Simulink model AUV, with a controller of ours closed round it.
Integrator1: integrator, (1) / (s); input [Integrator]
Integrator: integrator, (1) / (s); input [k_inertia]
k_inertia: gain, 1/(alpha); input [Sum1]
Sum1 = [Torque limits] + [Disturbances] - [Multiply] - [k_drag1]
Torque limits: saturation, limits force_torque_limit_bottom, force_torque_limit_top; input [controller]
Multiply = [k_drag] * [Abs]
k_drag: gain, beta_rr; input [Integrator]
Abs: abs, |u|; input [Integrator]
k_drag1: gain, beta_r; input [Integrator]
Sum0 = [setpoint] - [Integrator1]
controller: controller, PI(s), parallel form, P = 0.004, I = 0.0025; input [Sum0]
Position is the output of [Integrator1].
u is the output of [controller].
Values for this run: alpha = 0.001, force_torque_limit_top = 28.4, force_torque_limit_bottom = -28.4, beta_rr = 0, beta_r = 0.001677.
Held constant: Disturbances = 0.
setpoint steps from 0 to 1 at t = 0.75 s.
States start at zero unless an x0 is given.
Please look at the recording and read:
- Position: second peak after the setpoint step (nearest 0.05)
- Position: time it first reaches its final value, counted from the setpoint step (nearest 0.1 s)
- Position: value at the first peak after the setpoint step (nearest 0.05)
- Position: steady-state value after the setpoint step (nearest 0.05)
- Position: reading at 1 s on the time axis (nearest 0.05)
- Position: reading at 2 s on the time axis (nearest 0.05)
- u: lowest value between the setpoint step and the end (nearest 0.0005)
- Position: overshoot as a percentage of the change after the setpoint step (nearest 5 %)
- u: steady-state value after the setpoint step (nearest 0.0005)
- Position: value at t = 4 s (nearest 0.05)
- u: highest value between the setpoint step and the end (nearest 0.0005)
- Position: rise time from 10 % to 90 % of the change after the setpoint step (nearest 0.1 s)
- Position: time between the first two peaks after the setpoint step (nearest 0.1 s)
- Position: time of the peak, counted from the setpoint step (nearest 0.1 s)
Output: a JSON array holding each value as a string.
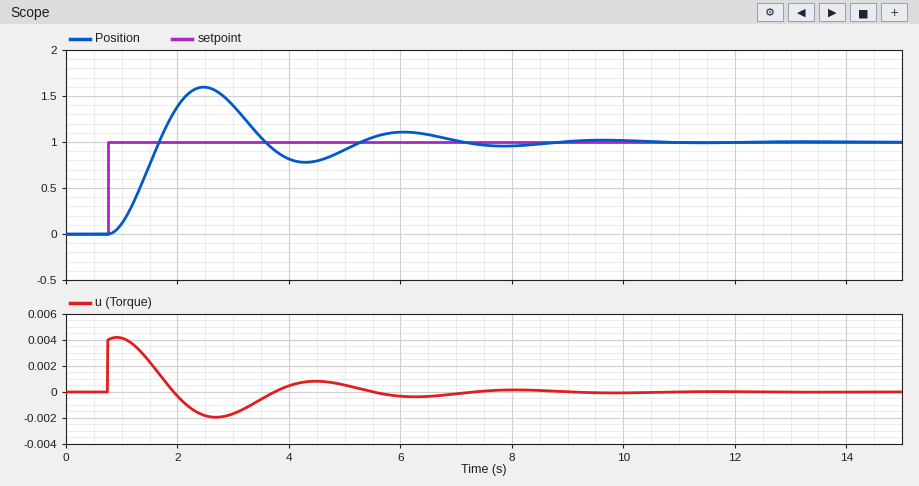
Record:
["1.10", "0.9 s", "1.60", "1.00", "0.10", "1.40", "-0.0020", "60 %", "0.0000", "0.80", "0.0040", "0.6 s", "3.6 s", "1.7 s"]
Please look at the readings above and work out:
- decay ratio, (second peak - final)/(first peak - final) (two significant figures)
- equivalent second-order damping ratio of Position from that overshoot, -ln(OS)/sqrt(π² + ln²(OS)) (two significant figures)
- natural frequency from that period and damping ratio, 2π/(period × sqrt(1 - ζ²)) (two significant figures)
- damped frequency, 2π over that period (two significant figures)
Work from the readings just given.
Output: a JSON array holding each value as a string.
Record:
["0.17", "0.16", "1.8 rad/s", "1.7 rad/s"]
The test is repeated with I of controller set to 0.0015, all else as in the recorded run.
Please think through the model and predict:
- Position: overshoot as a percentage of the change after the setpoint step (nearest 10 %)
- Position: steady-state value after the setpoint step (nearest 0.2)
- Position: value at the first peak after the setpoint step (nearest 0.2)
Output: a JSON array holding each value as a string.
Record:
["50 %", "1.0", "1.4"]
